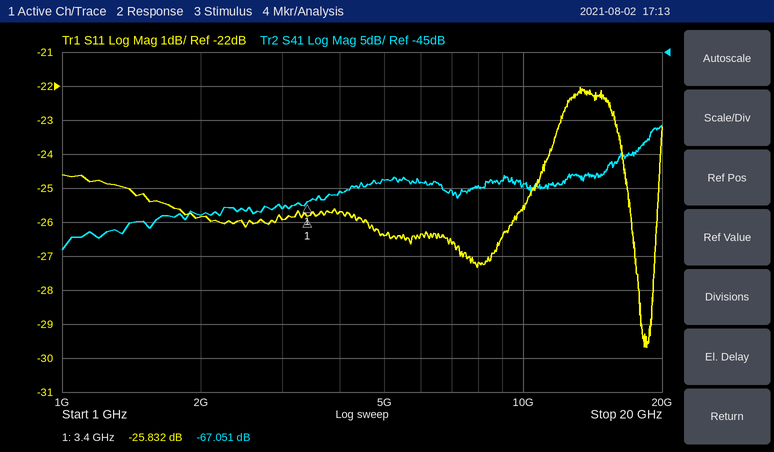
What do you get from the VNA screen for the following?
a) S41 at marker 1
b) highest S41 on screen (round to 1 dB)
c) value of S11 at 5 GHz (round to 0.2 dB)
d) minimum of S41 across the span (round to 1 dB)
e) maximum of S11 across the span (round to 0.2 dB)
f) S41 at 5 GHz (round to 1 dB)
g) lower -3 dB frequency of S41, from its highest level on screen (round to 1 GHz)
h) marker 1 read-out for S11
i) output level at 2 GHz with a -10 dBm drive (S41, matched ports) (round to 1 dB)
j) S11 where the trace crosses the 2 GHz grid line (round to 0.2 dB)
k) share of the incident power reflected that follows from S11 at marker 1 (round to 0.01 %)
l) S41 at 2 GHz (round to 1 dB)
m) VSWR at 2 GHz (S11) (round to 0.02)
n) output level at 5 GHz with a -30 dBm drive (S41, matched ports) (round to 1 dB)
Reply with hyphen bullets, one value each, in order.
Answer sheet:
- -67.051 dB
- -56 dB
- -26.4 dB
- -74 dB
- -22.0 dB
- -64 dB
- 18 GHz
- -25.832 dB
- -79 dBm
- -25.8 dB
- 0.26 %
- -69 dB
- 1.10
- -94 dBm
